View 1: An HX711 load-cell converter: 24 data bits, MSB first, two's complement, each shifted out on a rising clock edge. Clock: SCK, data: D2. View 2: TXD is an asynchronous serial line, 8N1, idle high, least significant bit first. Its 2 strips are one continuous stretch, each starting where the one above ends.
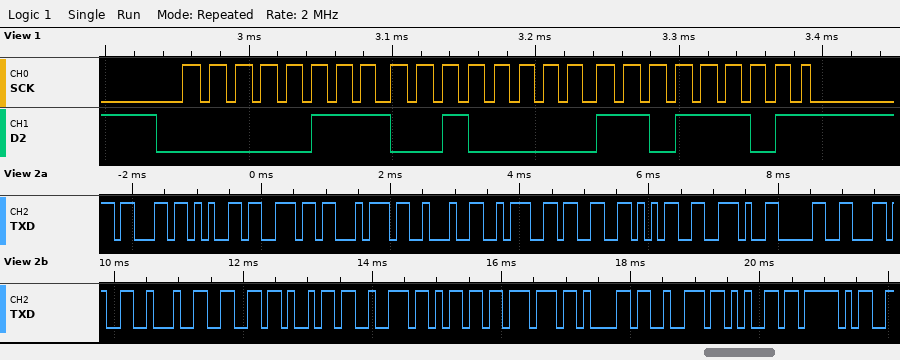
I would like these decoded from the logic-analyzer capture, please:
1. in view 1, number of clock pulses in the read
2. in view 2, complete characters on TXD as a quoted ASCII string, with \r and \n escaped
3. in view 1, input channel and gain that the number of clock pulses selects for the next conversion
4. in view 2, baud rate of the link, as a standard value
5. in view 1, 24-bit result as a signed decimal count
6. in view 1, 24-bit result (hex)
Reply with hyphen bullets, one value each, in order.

- 25
- "cent\":35.0,\"firmware_"
- channel A, gain 128
- 9600 baud
- 467165
- 0x0720DD
